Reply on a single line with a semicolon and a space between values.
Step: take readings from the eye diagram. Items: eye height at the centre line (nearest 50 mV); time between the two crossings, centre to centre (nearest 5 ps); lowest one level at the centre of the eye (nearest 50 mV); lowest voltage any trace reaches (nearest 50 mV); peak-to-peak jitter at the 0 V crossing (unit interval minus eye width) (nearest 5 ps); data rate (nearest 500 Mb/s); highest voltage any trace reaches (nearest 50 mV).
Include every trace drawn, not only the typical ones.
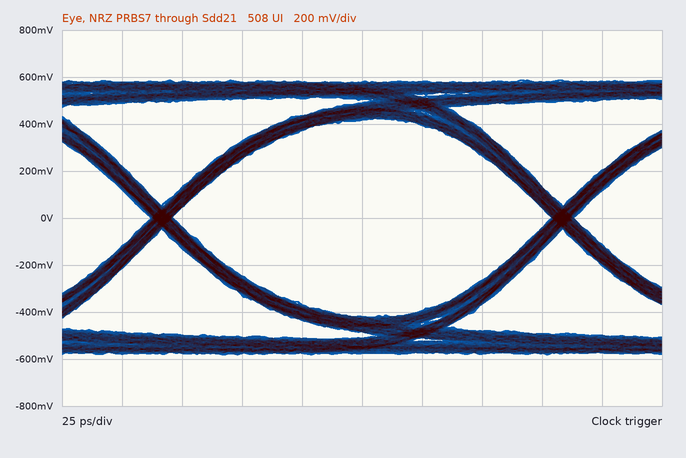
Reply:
850 mV; 165 ps; 400 mV; -600 mV; 10 ps; 6.0 Gb/s; 600 mV
